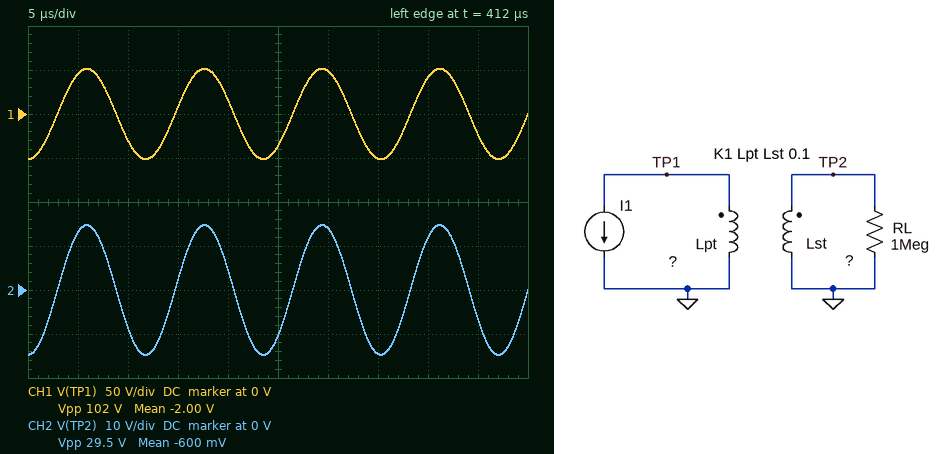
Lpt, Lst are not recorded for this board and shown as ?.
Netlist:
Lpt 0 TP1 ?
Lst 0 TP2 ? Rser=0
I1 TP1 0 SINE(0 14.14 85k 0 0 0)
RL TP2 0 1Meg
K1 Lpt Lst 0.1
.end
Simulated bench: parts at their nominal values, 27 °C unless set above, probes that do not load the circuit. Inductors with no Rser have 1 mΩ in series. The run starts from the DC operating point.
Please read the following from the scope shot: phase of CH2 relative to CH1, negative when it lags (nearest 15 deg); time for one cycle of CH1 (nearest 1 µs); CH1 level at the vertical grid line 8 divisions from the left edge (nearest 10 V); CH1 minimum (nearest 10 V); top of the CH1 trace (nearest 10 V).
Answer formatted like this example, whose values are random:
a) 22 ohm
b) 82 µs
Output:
a) 0 deg
b) 12 µs
c) 40 V
d) -50 V
e) 50 V
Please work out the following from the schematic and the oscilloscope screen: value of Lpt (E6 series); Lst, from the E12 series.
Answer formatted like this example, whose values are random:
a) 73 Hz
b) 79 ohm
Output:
a) 6.8 µH
b) 56 µH
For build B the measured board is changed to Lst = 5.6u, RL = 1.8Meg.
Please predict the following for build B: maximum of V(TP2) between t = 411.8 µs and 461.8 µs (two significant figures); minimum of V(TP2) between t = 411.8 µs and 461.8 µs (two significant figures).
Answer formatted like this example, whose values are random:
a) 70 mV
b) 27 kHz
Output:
a) 4.7 V
b) -4.7 V
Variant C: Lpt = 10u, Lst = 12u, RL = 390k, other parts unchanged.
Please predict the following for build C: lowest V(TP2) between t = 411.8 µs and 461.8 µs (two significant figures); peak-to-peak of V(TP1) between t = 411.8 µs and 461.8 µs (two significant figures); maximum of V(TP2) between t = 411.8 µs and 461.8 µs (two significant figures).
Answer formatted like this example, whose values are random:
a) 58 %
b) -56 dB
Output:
a) -8.3 V
b) 150 V
c) 8.3 V
